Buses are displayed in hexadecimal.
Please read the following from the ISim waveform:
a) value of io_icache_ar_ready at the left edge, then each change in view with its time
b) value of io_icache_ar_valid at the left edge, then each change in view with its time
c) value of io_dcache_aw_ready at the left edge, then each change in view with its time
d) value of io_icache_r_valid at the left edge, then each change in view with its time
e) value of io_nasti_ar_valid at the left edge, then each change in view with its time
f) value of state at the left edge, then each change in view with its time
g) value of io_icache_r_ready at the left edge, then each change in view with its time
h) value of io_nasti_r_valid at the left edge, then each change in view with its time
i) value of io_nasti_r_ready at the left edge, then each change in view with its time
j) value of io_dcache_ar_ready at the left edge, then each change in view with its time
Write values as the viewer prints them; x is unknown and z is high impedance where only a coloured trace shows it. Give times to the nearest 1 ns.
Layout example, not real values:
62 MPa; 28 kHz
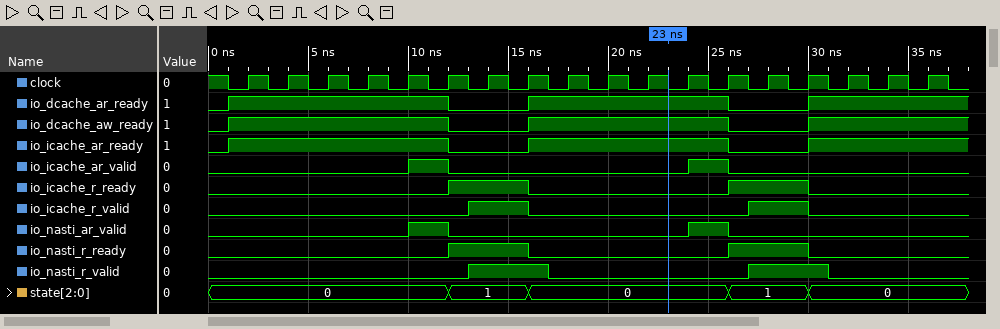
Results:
0, 1 at 1 ns, 0 at 12 ns, 1 at 16 ns, 0 at 26 ns, 1 at 30 ns; 0, 1 at 10 ns, 0 at 12 ns, 1 at 24 ns, 0 at 26 ns; 0, 1 at 1 ns, 0 at 12 ns, 1 at 16 ns, 0 at 26 ns, 1 at 30 ns; 0, 1 at 13 ns, 0 at 16 ns, 1 at 27 ns, 0 at 30 ns; 0, 1 at 10 ns, 0 at 12 ns, 1 at 24 ns, 0 at 26 ns; 0, 1 at 12 ns, 0 at 16 ns, 1 at 26 ns, 0 at 30 ns; 0, 1 at 12 ns, 0 at 16 ns, 1 at 26 ns, 0 at 30 ns; 0, 1 at 13 ns, 0 at 17 ns, 1 at 27 ns, 0 at 31 ns; 0, 1 at 12 ns, 0 at 16 ns, 1 at 26 ns, 0 at 30 ns; 0, 1 at 1 ns, 0 at 12 ns, 1 at 16 ns, 0 at 26 ns, 1 at 30 ns
